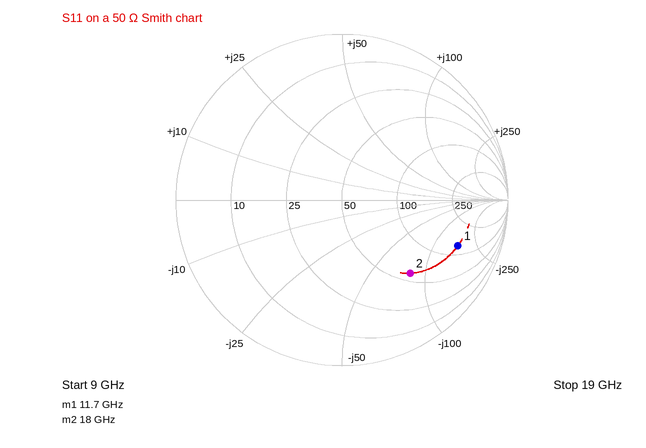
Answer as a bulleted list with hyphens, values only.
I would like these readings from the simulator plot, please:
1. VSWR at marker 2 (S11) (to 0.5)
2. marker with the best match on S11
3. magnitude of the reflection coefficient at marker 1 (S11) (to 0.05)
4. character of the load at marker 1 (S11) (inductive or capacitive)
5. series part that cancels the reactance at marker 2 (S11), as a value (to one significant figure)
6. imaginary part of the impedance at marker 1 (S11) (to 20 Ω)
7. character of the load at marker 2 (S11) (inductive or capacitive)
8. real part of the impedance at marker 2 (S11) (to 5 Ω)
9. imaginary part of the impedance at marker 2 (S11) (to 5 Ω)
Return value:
- 4.0
- marker 2
- 0.75
- capacitive
- 700 pH
- -160 Ω
- capacitive
- 60 Ω
- -80 Ω
